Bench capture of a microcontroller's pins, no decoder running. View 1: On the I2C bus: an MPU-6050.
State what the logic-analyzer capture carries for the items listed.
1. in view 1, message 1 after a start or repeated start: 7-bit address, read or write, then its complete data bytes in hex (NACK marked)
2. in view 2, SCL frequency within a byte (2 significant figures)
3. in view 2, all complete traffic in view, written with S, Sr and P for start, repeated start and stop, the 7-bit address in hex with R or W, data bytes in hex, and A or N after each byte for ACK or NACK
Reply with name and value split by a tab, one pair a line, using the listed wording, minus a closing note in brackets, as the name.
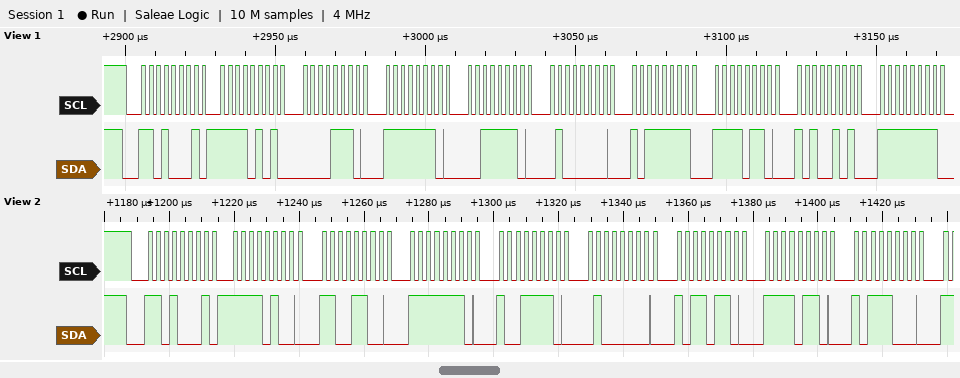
in view 1, message 1 after a start or repeated start: 7-bit address, read or write, then its complete data bytes in hex	0x68 read: F5 0E FE 3E 40 BF F6 A5 FF
in view 2, SCL frequency within a byte	400 kHz
in view 2, all complete traffic in view, written with S, Sr and P for start, repeated start and stop, the 7-bit address in hex with R or W, data bytes in hex, and A or N after each byte for ACK or NACK	S 68R A F4 A CC A FE A 9E A 40 A B6 A F6 A B8 A
